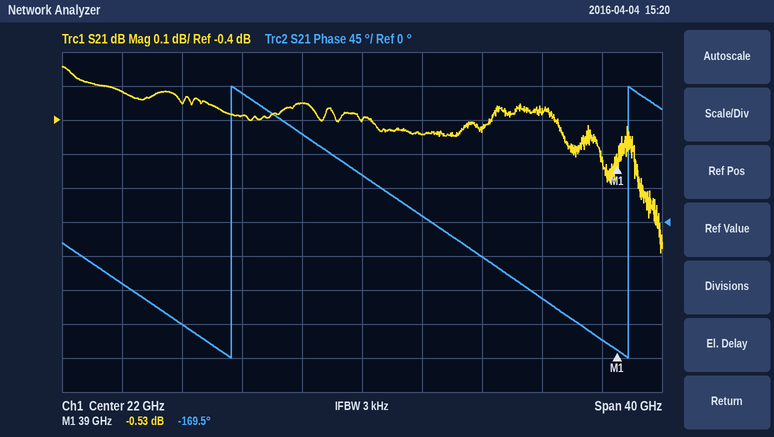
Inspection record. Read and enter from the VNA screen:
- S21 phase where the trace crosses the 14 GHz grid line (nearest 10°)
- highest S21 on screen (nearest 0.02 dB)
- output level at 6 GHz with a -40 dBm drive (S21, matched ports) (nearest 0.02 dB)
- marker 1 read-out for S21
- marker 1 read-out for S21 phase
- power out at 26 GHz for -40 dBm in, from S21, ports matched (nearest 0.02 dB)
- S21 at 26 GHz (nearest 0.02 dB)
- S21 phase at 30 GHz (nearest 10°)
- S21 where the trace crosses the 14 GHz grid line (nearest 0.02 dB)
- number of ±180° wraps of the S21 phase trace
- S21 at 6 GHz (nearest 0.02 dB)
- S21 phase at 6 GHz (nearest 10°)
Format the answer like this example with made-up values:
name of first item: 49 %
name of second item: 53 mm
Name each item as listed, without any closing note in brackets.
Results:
S21 phase where the trace crosses the 14 GHz grid line: 170°
highest S21 on screen: -0.24 dB
output level at 6 GHz with a -40 dBm drive (S21, matched ports): -40.32 dBm
marker 1 read-out for S21: -0.53 dB
marker 1 read-out for S21 phase: -169.5°
power out at 26 GHz for -40 dBm in, from S21, ports matched: -40.44 dBm
S21 at 26 GHz: -0.44 dB
S21 phase at 30 GHz: -50°
S21 where the trace crosses the 14 GHz grid line: -0.38 dB
number of ±180° wraps of the S21 phase trace: 2
S21 at 6 GHz: -0.32 dB
S21 phase at 6 GHz: -80°
